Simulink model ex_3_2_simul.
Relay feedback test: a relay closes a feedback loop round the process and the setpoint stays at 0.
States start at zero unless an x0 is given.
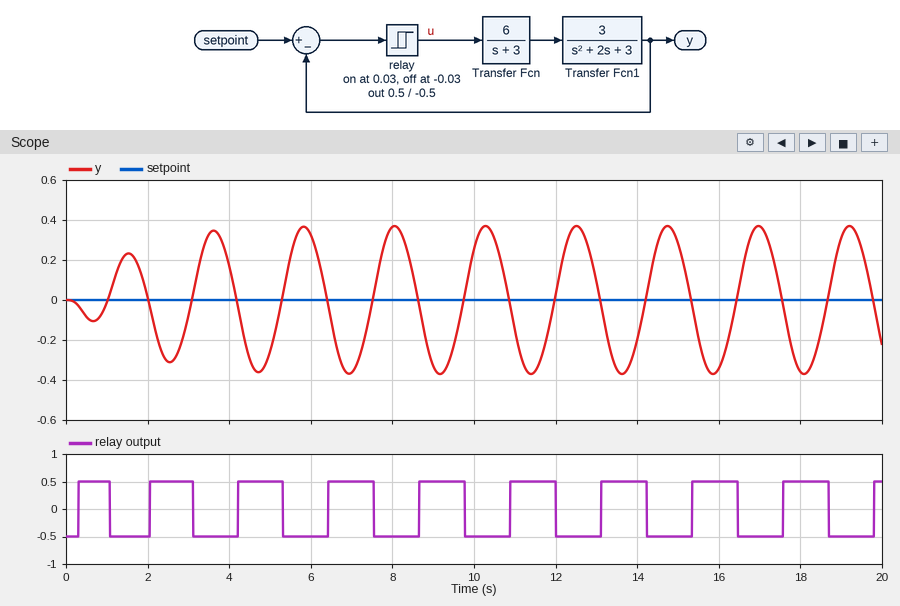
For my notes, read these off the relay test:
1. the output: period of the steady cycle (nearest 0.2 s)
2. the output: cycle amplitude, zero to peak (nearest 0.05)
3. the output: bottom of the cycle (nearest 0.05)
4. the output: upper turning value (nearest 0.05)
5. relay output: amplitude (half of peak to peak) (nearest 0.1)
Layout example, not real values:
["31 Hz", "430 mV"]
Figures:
["2.2 s", "0.35", "-0.35", "0.35", "0.5"]
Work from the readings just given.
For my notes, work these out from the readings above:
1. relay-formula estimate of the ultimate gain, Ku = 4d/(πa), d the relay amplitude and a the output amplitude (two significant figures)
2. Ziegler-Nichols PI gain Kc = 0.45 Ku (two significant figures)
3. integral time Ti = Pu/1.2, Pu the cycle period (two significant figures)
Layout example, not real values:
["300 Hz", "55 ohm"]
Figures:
["1.8", "0.81", "1.8 s"]
